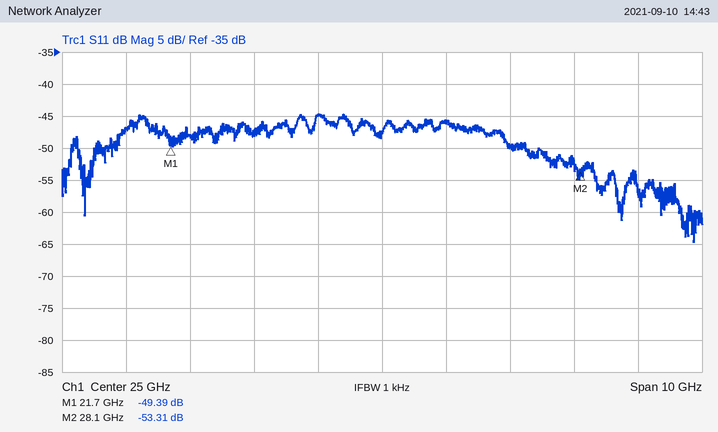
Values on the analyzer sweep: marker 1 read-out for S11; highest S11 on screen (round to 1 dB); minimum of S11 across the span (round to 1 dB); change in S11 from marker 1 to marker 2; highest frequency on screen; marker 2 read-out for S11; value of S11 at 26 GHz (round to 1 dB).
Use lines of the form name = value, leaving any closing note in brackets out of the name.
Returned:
marker 1 read-out for S11 = -49.39 dB
highest S11 on screen = -45 dB
minimum of S11 across the span = -65 dB
change in S11 from marker 1 to marker 2 = -3.92 dB
highest frequency on screen = 30 GHz
marker 2 read-out for S11 = -53.31 dB
value of S11 at 26 GHz = -46 dB
